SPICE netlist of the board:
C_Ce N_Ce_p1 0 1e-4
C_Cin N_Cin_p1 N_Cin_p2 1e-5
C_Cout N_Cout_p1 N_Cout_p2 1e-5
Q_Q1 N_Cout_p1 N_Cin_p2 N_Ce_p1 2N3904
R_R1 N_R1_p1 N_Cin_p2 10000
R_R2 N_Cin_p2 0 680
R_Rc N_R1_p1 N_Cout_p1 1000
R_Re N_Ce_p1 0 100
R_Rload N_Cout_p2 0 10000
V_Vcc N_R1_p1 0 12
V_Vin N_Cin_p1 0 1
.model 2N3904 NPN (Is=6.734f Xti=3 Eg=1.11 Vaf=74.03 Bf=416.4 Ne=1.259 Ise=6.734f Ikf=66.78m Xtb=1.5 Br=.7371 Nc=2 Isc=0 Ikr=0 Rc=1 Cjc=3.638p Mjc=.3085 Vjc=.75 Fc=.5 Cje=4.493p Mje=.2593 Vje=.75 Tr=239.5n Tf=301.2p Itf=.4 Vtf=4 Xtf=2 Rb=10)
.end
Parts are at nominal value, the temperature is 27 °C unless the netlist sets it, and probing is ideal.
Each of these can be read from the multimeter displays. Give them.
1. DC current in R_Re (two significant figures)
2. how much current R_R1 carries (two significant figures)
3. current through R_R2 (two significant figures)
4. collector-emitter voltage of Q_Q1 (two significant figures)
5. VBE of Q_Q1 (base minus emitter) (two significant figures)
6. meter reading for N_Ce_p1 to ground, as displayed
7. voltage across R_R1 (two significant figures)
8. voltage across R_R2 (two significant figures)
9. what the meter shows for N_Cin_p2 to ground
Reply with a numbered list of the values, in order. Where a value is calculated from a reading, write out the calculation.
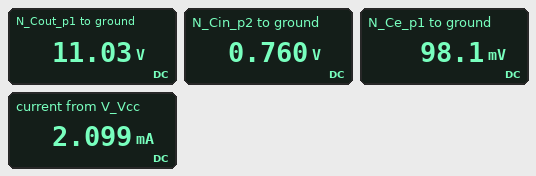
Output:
1. (98.1 mV) / 100 Ω = 980 µA
2. (12 V - 760 mV) / 10 kΩ = 1.1 mA
3. (760 mV) / 680 Ω = 1.1 mA
4. 11.03 V - 98.1 mV = 11 V
5. 760 mV - 98.1 mV = 660 mV
6. 98.1 mV
7. 12 V - 760 mV = 11 V
8. 760 mV = 760 mV
9. 0.760 V
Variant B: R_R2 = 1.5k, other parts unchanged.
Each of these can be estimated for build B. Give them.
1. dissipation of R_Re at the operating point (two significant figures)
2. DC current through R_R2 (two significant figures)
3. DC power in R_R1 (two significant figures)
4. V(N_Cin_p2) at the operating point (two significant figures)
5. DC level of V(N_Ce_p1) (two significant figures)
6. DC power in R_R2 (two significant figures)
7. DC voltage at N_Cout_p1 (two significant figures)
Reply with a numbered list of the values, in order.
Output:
1. 6.1 mW
2. 1.0 mA
3. 11 mW
4. 1.5 V
5. 780 mV
6. 1.5 mW
7. 4.2 V
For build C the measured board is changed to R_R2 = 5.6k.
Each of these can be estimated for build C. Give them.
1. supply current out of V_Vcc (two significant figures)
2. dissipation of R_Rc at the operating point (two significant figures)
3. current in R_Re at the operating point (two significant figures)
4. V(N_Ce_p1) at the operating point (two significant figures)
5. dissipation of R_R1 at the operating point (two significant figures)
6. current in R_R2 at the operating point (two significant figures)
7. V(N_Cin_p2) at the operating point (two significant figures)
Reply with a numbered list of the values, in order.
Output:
1. 12 mA
2. 120 mW
3. 11 mA
4. 1.1 V
5. 10 mW
6. 340 µA
7. 1.9 V
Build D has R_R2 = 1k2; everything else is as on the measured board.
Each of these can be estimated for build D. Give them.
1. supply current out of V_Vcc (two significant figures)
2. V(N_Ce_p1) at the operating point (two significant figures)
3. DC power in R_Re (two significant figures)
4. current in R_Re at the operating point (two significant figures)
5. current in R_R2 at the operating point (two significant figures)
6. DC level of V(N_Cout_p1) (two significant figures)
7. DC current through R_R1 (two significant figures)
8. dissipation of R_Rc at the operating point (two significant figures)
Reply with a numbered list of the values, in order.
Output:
1. 6.5 mA
2. 540 mV
3. 2.9 mW
4. 5.4 mA
5. 1.0 mA
6. 6.6 V
7. 1.1 mA
8. 29 mW
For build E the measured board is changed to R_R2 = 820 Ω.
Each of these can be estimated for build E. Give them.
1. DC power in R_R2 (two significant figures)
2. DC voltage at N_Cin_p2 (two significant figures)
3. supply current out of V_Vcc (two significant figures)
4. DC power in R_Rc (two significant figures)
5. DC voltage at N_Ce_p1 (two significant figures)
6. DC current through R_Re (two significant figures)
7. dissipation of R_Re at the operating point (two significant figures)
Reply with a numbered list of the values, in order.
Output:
1. 990 µW
2. 900 mV
3. 3.3 mA
4. 4.6 mW
5. 220 mV
6. 2.2 mA
7. 470 µW
